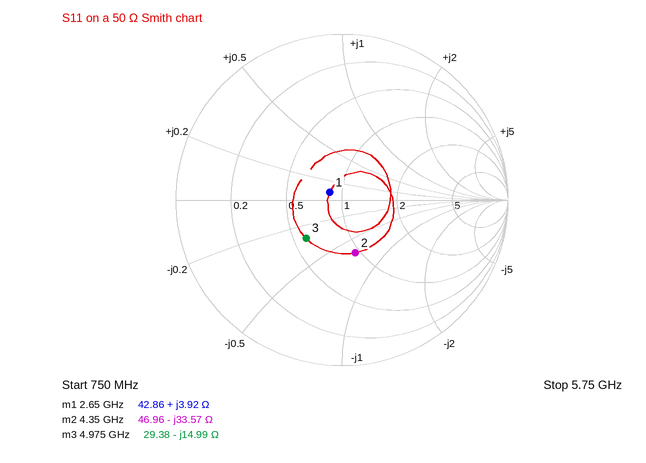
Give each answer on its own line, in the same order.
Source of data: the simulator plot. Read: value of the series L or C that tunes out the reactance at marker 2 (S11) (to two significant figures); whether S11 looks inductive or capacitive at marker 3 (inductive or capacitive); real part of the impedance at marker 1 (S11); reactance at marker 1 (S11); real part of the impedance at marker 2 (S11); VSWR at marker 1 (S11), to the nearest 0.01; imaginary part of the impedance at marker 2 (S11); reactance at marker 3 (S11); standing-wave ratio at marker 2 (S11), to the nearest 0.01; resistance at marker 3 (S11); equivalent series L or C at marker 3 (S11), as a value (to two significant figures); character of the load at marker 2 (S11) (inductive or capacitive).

1.2 nH
capacitive
42.86 Ω
+3.92 Ω
46.96 Ω
1.19
-33.57 Ω
-14.99 Ω
1.98
29.38 Ω
2.1 pF
capacitive
